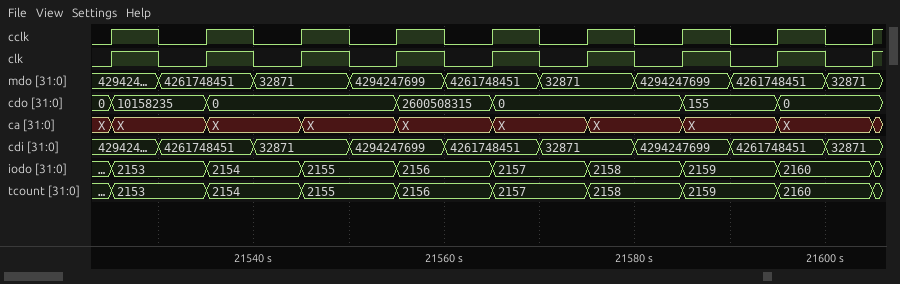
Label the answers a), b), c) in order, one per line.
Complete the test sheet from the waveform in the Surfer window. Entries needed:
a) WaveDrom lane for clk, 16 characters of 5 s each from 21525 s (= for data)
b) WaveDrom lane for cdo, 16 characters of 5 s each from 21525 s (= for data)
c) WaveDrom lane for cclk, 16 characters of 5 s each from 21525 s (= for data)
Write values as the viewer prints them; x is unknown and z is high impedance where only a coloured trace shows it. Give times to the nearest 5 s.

a) {name: 'clk', wave: '1010101010101010'}
b) {name: 'cdo', wave: '=.=...=.=...=.=.', data: '10158235 0 2600508315 0 155 0'}
c) {name: 'cclk', wave: '1010101010101010'}
